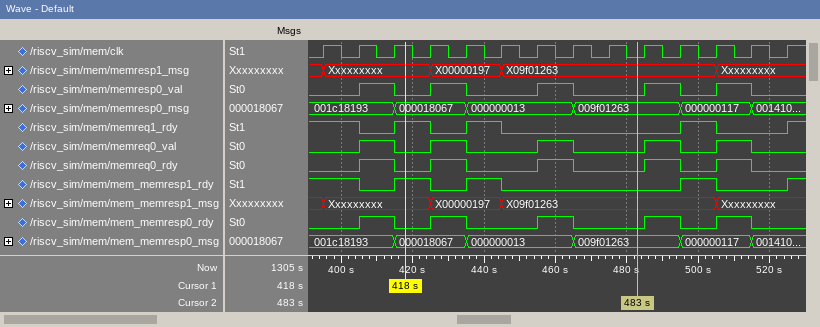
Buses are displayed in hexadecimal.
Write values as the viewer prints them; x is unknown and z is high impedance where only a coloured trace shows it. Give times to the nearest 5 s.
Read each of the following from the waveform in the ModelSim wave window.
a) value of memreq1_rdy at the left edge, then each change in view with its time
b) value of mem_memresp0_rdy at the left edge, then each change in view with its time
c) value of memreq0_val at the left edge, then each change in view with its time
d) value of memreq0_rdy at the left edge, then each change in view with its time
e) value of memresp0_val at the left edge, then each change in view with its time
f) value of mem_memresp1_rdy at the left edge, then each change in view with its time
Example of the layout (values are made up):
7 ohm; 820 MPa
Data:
1, 0 at 405 s, 1 at 415 s, 0 at 425 s, 1 at 435 s, 0 at 445 s, 1 at 495 s, 0 at 505 s, 1 at 525 s; 0, 1 at 405 s, 0 at 415 s, 1 at 425 s, 0 at 435 s, 1 at 455 s, 0 at 465 s, 1 at 485 s, 0 at 495 s, 1 at 505 s, 0 at 515 s; 0, 1 at 405 s, 0 at 415 s, 1 at 425 s, 0 at 435 s, 1 at 455 s, 0 at 465 s, 1 at 485 s, 0 at 495 s, 1 at 505 s, 0 at 515 s; 0, 1 at 405 s, 0 at 415 s, 1 at 425 s, 0 at 435 s, 1 at 455 s, 0 at 465 s, 1 at 485 s, 0 at 495 s, 1 at 505 s, 0 at 515 s; 0, 1 at 405 s, 0 at 415 s, 1 at 425 s, 0 at 435 s, 1 at 455 s, 0 at 465 s, 1 at 485 s, 0 at 495 s, 1 at 505 s, 0 at 515 s; 1, 0 at 405 s, 1 at 415 s, 0 at 425 s, 1 at 435 s, 0 at 445 s, 1 at 495 s, 0 at 505 s, 1 at 525 s
